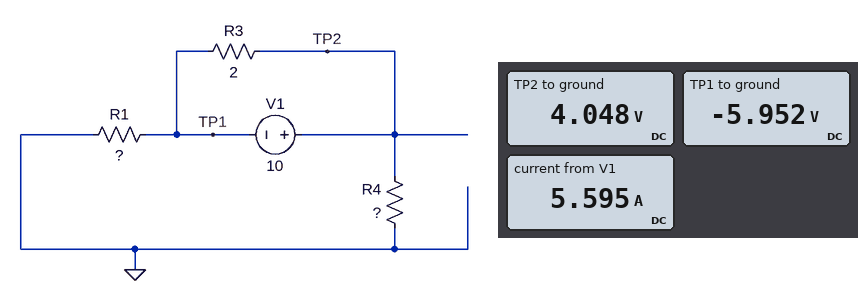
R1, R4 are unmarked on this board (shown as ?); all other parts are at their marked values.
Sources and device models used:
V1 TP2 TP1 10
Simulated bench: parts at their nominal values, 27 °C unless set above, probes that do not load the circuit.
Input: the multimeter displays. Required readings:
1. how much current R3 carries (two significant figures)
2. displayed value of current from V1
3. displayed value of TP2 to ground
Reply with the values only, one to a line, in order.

5.0 A
5.595 A
4.048 V
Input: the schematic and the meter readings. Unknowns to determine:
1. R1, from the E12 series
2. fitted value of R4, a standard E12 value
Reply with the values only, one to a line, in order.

10 Ω
6.8 Ω
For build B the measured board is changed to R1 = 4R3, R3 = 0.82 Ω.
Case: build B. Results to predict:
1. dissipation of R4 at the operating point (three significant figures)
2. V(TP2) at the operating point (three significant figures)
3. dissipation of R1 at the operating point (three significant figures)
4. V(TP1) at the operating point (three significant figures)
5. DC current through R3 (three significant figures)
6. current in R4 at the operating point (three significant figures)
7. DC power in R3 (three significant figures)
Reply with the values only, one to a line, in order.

5.52 W
6.13 V
3.49 W
-3.87 V
12.2 A
901 mA
122 W
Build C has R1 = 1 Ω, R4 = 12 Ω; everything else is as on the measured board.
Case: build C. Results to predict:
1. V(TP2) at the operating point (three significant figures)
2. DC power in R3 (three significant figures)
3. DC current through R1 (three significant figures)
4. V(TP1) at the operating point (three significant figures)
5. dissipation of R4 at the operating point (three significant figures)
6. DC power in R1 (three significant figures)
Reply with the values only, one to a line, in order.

9.23 V
50.0 W
769 mA
-769 mV
7.10 W
592 mW
